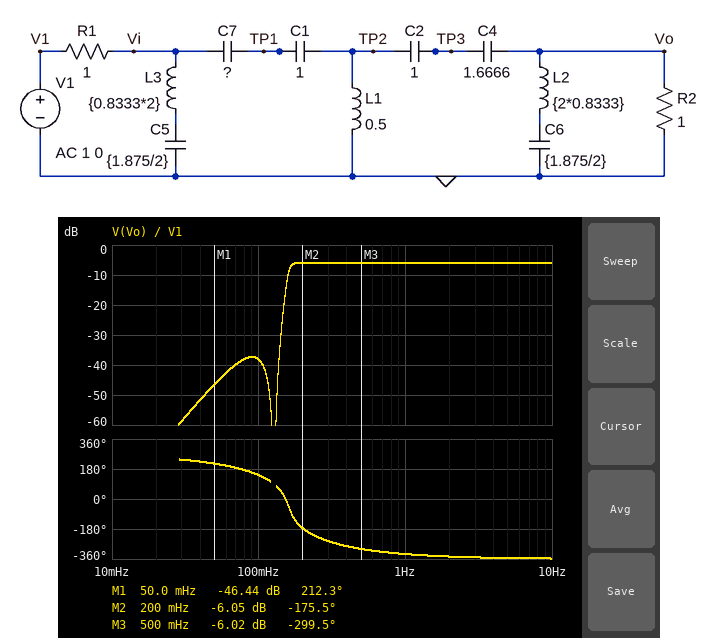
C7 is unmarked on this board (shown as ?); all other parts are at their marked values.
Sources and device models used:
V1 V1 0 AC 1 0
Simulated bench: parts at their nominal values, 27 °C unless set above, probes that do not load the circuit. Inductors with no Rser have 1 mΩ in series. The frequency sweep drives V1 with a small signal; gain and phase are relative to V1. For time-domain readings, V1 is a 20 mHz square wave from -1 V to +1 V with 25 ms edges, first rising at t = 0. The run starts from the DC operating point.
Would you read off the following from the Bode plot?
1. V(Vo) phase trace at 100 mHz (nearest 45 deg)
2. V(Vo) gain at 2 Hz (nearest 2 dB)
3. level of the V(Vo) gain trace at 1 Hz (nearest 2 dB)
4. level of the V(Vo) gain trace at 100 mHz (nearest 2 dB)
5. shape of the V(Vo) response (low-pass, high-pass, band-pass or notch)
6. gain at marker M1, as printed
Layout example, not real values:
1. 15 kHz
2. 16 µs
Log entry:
1. 135 deg
2. -6 dB
3. -6 dB
4. -38 dB
5. high-pass
6. -46.44 dB
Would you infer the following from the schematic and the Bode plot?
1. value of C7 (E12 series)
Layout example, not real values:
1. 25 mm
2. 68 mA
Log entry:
1. 1.5 F
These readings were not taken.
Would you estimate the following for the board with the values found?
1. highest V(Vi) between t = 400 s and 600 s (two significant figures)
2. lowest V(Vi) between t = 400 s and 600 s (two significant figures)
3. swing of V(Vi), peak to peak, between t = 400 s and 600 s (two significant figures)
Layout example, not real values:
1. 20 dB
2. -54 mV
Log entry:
1. 1.2 V
2. -1.2 V
3. 2.4 V
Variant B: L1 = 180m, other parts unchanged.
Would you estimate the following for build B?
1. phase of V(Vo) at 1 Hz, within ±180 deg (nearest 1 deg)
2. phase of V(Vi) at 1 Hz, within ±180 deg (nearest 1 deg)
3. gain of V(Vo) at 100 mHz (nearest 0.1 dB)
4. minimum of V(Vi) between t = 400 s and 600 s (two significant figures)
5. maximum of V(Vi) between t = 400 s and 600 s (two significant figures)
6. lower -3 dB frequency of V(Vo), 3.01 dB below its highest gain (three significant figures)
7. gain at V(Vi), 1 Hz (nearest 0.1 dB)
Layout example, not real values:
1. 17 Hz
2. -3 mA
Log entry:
1. 46 deg
2. 13 deg
3. -48.3 dB
4. -1.3 V
5. 1.3 V
6. 334 mHz
7. -7.7 dB
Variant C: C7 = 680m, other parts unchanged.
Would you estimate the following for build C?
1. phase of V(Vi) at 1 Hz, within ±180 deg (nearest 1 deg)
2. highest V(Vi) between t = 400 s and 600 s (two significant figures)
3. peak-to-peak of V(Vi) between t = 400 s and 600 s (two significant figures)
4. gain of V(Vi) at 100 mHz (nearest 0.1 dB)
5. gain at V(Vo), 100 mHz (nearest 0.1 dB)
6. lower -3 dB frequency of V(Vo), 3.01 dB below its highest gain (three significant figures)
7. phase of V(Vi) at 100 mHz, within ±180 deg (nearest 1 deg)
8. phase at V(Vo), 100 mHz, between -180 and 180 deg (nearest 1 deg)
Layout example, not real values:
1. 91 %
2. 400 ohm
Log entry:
1. -4 deg
2. 1.2 V
3. 2.5 V
4. -6.3 dB
5. -41.4 dB
6. 177 mHz
7. -61 deg
8. 145 deg
